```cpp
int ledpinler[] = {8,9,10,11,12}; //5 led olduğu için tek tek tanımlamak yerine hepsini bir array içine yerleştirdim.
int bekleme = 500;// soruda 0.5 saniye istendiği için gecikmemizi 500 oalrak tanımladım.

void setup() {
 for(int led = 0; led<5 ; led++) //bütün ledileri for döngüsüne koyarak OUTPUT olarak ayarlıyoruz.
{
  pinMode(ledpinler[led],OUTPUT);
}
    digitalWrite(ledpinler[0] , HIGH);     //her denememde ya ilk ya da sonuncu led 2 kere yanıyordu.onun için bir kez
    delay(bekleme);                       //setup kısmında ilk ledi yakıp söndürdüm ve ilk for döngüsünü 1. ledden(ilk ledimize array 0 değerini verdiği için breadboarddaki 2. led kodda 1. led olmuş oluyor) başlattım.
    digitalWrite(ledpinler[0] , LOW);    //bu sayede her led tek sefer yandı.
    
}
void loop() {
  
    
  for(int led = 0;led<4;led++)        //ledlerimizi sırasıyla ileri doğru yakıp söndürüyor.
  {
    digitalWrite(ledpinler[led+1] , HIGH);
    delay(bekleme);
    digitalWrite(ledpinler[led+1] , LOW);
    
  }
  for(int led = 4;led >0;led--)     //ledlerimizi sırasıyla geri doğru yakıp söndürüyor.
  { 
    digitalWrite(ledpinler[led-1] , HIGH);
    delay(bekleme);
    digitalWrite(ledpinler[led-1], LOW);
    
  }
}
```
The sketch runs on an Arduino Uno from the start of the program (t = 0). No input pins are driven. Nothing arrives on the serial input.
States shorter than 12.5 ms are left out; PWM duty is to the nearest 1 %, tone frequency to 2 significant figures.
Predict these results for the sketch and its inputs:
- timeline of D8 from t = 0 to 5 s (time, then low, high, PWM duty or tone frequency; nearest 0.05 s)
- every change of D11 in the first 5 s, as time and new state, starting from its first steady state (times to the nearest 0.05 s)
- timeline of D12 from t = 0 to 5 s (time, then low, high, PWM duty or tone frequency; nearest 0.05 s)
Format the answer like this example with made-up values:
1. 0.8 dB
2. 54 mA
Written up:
1. 0 s high; 0.5 s low; 4 s high; 4.5 s low
2. 0 s low; 1.5 s high; 2 s low; 2.5 s high; 3 s low
3. 0 s low; 2 s high; 2.5 s low
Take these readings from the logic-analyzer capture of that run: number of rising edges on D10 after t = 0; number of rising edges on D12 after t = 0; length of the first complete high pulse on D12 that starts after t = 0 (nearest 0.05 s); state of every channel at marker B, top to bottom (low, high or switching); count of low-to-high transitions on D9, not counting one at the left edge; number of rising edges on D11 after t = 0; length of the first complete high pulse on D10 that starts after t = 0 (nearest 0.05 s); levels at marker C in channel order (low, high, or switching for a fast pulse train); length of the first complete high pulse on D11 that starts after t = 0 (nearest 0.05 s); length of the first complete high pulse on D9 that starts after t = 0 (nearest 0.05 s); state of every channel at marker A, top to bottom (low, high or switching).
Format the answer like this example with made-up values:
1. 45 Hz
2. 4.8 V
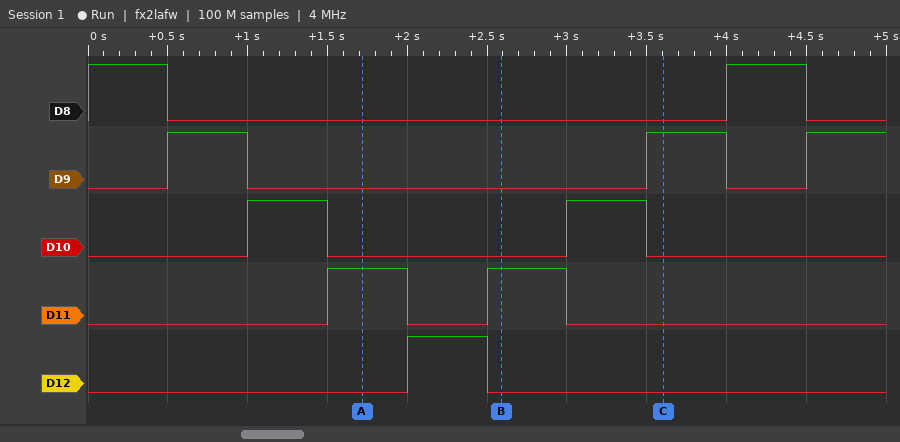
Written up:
1. 2
2. 1
3. 0.50 s
4. D8 low, D9 low, D10 low, D11 high, D12 low
5. 3
6. 2
7. 0.50 s
8. D8 low, D9 high, D10 low, D11 low, D12 low
9. 0.50 s
10. 0.50 s
11. D8 low, D9 low, D10 low, D11 high, D12 low
